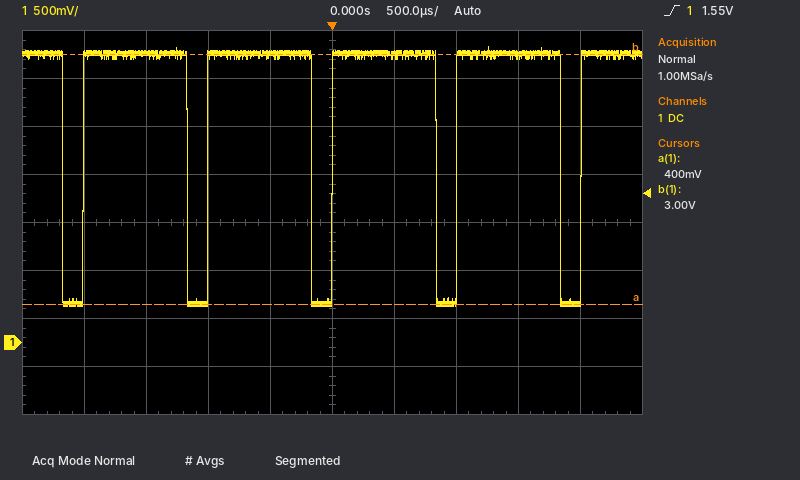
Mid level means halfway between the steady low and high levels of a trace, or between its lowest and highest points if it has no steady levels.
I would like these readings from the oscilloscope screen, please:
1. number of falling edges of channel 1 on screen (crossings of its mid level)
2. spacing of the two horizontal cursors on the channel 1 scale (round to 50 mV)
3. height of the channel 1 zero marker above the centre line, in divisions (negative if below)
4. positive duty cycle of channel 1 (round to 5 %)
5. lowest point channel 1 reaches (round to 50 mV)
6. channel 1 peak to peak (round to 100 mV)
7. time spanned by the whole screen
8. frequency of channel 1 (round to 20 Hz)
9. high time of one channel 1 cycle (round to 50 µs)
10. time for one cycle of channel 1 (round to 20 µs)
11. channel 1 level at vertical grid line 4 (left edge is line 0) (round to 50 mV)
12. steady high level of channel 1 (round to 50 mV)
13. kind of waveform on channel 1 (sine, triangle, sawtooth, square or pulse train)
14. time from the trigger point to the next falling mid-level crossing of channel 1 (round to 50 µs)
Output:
5
2.60 V
-2.5 div
85 %
400 mV
2.70 V
5 ms
1.00 kHz
850 µs
1.00 ms
3.00 V
3.00 V
pulse train
850 µs
